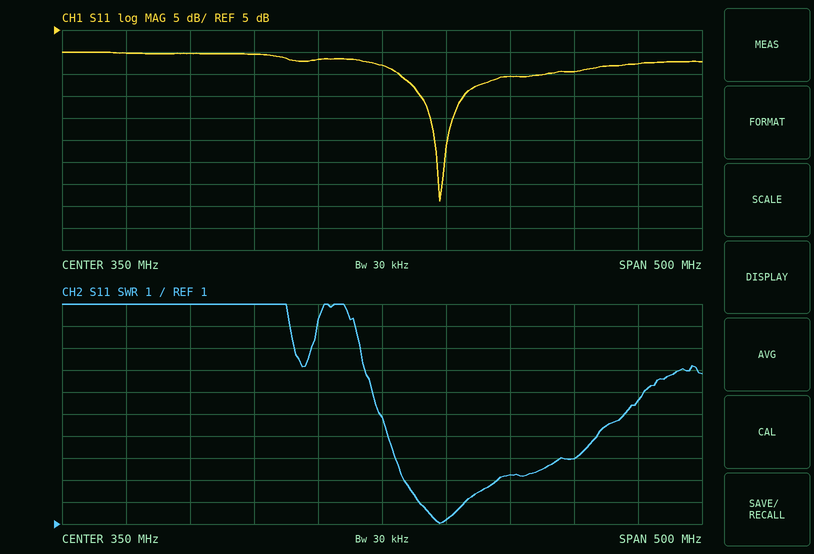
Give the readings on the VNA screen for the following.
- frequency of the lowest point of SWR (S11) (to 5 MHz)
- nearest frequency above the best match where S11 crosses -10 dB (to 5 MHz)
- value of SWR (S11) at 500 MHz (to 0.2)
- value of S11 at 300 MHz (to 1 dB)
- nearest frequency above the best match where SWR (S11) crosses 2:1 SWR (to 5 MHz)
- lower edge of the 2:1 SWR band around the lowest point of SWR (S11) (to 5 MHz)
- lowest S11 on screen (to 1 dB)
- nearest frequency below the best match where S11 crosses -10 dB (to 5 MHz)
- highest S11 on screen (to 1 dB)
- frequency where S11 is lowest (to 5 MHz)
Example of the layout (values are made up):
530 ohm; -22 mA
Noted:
395 MHz; 415 MHz; 4.0; -2 dB; 415 MHz; 380 MHz; -34 dB; 380 MHz; 0 dB; 395 MHz
